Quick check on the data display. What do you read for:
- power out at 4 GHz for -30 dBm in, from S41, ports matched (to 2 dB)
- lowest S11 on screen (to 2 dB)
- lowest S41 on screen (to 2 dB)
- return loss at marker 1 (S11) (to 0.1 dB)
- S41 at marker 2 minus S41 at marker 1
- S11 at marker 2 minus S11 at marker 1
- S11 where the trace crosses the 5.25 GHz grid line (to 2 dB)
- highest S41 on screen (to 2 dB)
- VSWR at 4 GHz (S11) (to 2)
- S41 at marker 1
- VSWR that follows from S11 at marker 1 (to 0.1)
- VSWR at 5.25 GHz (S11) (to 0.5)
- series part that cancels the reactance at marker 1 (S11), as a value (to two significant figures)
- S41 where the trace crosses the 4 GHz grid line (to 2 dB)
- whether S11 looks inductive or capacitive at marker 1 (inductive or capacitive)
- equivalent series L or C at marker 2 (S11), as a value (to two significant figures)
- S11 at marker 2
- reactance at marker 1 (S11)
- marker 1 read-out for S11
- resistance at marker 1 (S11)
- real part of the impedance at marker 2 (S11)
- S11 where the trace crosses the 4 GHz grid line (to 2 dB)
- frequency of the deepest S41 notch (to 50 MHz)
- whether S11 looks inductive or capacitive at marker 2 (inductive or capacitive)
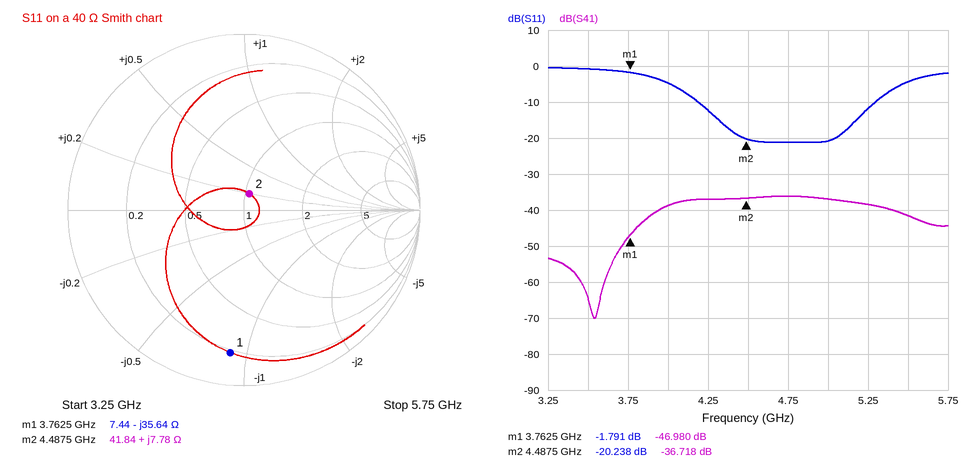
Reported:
-68 dBm
-22 dB
-70 dB
1.8 dB
10.262 dB
-18.447 dB
-12 dB
-36 dB
4
-46.980 dB
9.7
1.5
1.5 nH
-38 dB
capacitive
280 pH
-20.238 dB
-35.64 Ω
-1.791 dB
7.44 Ω
41.84 Ω
-4 dB
3.55 GHz
inductive
